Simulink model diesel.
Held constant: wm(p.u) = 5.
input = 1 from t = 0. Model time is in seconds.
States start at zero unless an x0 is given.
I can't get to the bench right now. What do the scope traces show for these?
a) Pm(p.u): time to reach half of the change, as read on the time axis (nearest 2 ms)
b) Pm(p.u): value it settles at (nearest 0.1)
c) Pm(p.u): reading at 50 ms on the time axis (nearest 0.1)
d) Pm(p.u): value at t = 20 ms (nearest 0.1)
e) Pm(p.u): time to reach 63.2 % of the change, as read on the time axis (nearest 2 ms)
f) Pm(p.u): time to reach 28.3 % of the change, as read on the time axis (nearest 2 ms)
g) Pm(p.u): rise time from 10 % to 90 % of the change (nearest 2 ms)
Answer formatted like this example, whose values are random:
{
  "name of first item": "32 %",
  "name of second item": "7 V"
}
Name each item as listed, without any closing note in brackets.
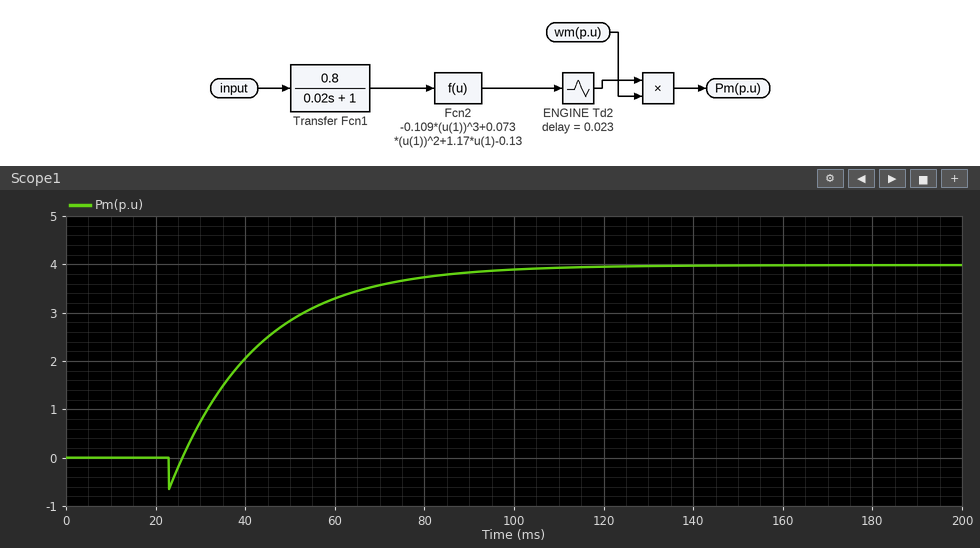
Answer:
{
  "Pm(p.u): time to reach half of the change, as read on the time axis": "40 ms",
  "Pm(p.u): value it settles at": "4.0",
  "Pm(p.u): reading at 50 ms on the time axis": "2.8",
  "Pm(p.u): value at t = 20 ms": "0.0",
  "Pm(p.u): time to reach 63.2 % of the change, as read on the time axis": "46 ms",
  "Pm(p.u): time to reach 28.3 % of the change, as read on the time axis": "32 ms",
  "Pm(p.u): rise time from 10 % to 90 % of the change": "42 ms"
}
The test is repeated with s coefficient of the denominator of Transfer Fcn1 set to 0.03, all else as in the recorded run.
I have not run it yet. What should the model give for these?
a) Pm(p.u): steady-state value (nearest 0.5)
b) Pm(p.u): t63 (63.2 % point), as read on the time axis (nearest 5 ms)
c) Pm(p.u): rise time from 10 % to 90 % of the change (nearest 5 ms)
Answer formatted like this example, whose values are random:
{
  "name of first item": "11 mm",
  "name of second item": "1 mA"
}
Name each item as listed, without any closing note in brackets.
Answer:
{
  "Pm(p.u): steady-state value": "4.0",
  "Pm(p.u): t63 (63.2 % point), as read on the time axis": "55 ms",
  "Pm(p.u): rise time from 10 % to 90 % of the change": "65 ms"
}
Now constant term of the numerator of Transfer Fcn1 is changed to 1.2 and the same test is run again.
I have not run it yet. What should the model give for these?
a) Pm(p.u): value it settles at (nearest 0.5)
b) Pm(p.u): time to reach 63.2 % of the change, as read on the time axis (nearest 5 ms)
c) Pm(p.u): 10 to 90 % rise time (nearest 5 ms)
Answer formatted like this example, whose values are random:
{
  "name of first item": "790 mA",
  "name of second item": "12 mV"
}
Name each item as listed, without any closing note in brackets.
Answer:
{
  "Pm(p.u): value it settles at": "6.0",
  "Pm(p.u): time to reach 63.2 % of the change, as read on the time axis": "45 ms",
  "Pm(p.u): 10 to 90 % rise time": "40 ms"
}
